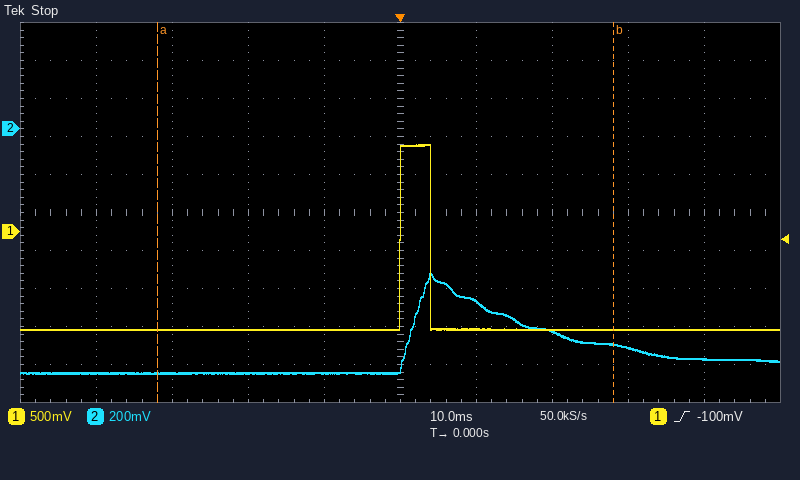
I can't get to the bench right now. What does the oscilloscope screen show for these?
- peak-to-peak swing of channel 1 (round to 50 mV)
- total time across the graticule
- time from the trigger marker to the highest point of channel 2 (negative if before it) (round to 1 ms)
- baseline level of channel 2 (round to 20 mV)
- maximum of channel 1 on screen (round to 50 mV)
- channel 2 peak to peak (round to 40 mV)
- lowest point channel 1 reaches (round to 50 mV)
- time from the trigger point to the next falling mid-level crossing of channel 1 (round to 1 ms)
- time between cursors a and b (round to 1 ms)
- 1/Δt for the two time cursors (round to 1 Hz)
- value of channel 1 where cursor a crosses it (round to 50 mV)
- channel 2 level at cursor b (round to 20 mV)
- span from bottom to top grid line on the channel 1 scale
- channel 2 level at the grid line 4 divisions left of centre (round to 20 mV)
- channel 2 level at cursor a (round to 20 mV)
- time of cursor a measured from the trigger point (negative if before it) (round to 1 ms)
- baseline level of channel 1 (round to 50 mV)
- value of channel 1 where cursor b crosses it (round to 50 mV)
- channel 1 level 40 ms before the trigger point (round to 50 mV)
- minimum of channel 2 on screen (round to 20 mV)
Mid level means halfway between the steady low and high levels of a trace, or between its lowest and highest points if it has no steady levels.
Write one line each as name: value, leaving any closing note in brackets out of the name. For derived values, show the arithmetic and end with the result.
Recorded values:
peak-to-peak swing of channel 1: 1.15 V − (-1.30 V) = 2.45 V
total time across the graticule: 100 ms
time from the trigger marker to the highest point of channel 2 (negative if before it): +4 ms
baseline level of channel 2: -1.28 V
maximum of channel 1 on screen: 1.15 V
channel 2 peak to peak: 520 mV
lowest point channel 1 reaches: -1.30 V
time from the trigger point to the next falling mid-level crossing of channel 1: 4 ms
time between cursors a and b: 60 ms
1/Δt for the two time cursors: 1 / 60 ms ≈ 17 Hz
value of channel 1 where cursor a crosses it: -1.30 V
channel 2 level at cursor b: -1.14 V
span from bottom to top grid line on the channel 1 scale: 5 V
channel 2 level at the grid line 4 divisions left of centre: -1.28 V
channel 2 level at cursor a: -1.28 V
time of cursor a measured from the trigger point (negative if before it): -32 ms
baseline level of channel 1: -1.30 V
value of channel 1 where cursor b crosses it: -1.30 V
channel 1 level 40 ms before the trigger point: -1.30 V
minimum of channel 2 on screen: -1.28 V
